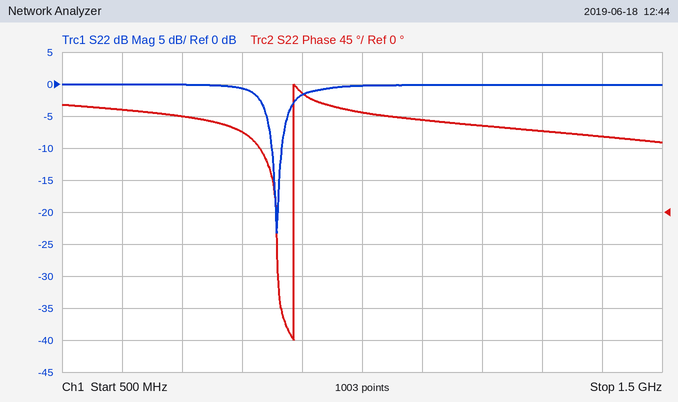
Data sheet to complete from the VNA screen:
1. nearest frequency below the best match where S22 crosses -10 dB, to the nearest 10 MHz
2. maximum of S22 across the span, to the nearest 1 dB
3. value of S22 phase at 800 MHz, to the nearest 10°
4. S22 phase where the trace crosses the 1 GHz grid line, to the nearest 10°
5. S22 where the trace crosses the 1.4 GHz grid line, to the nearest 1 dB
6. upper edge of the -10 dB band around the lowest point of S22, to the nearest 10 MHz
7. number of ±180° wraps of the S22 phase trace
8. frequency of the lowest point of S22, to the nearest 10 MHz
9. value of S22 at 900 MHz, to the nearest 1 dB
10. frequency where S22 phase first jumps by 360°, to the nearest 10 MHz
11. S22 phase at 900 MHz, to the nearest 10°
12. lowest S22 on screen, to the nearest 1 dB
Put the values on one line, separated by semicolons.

850 MHz; 0 dB; 110°; 140°; 0 dB; 870 MHz; 1; 860 MHz; -2 dB; 890 MHz; 170°; -23 dB
